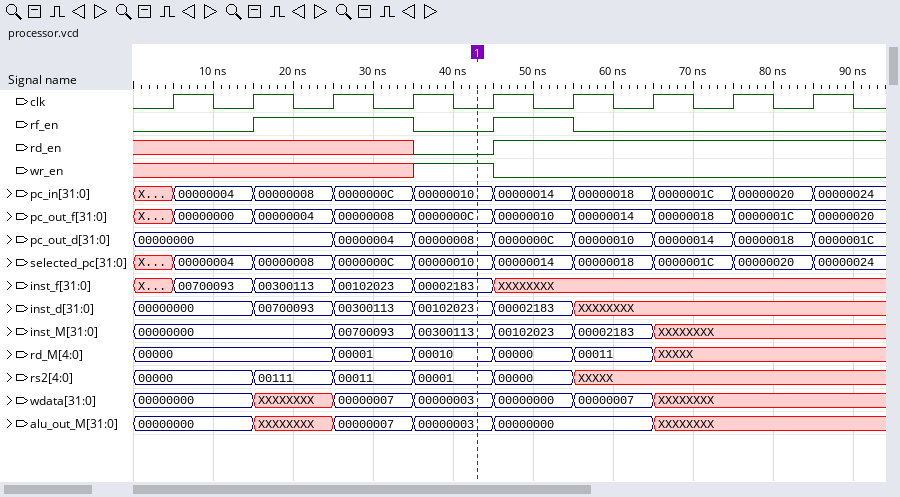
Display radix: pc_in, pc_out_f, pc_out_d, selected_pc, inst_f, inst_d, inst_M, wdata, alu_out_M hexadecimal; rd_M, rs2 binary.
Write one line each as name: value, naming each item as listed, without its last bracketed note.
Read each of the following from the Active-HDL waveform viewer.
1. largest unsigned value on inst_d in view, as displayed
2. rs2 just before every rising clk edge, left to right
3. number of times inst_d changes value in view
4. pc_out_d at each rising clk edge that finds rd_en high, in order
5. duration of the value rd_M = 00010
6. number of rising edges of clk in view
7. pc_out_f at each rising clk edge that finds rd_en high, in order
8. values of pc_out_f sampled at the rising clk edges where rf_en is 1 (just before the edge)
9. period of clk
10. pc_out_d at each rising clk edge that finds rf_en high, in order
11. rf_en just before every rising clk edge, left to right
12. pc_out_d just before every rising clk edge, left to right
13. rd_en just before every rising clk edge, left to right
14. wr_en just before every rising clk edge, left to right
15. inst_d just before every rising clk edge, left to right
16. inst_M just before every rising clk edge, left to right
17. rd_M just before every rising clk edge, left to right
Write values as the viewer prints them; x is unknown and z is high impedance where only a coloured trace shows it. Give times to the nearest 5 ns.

largest unsigned value on inst_d in view, as displayed: 00700093
rs2 just before every rising clk edge, left to right: 00000, 00000, 00111, 00011, 00001, 00000, XXXXX, XXXXX, XXXXX
number of times inst_d changes value in view: 5
pc_out_d at each rising clk edge that finds rd_en high, in order: 0000000C, 00000010, 00000014, 00000018
duration of the value rd_M = 00010: 10 ns
number of rising edges of clk in view: 9
pc_out_f at each rising clk edge that finds rd_en high, in order: 00000010, 00000014, 00000018, 0000001C
values of pc_out_f sampled at the rising clk edges where rf_en is 1: 00000004, 00000008, 00000010
period of clk: 10 ns
pc_out_d at each rising clk edge that finds rf_en high, in order: 00000000, 00000004, 0000000C
rf_en just before every rising clk edge, left to right: 0 0 1 1 0 1 0 0 0
pc_out_d just before every rising clk edge, left to right: 00000000, 00000000, 00000000, 00000004, 00000008, 0000000C, 00000010, 00000014, 00000018
rd_en just before every rising clk edge, left to right: x x x x 0 1 1 1 1
wr_en just before every rising clk edge, left to right: x x x x 1 0 0 0 0
inst_d just before every rising clk edge, left to right: 00000000, 00000000, 00700093, 00300113, 00102023, 00002183, XXXXXXXX, XXXXXXXX, XXXXXXXX
inst_M just before every rising clk edge, left to right: 00000000, 00000000, 00000000, 00700093, 00300113, 00102023, 00002183, XXXXXXXX, XXXXXXXX
rd_M just before every rising clk edge, left to right: 00000, 00000, 00000, 00001, 00010, 00000, 00011, XXXXX, XXXXX
